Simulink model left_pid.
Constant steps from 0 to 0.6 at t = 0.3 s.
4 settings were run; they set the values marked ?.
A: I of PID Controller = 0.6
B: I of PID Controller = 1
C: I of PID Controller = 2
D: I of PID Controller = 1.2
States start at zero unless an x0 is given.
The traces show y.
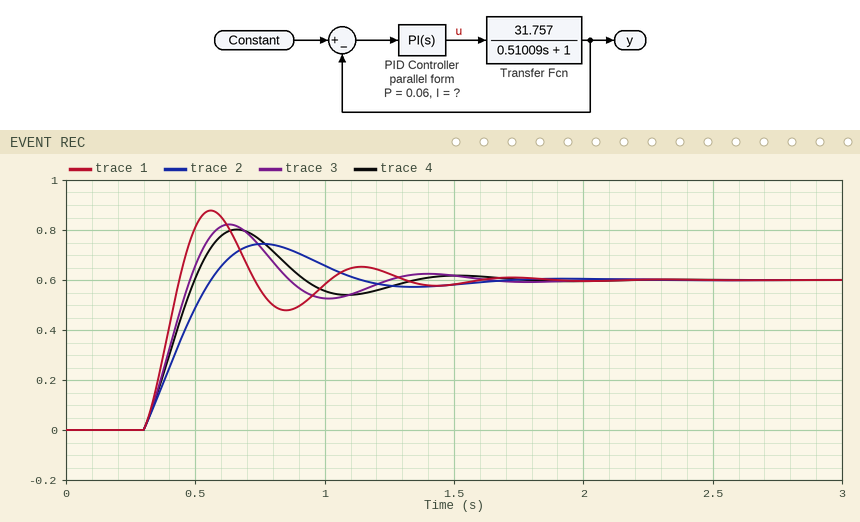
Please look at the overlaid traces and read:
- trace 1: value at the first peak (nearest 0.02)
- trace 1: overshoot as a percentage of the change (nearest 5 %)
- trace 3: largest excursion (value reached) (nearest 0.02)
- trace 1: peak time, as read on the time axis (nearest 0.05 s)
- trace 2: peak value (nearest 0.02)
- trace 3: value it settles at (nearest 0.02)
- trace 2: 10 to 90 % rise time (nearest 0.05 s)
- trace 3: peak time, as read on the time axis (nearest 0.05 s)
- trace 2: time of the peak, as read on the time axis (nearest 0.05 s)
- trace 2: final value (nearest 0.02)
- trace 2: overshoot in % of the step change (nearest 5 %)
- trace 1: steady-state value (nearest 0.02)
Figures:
0.88
45 %
0.82
0.55 s
0.74
0.60
0.20 s
0.65 s
0.75 s
0.60
25 %
0.60
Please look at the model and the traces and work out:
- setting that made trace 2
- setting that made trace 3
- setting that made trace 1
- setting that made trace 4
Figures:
A
D
C
B
